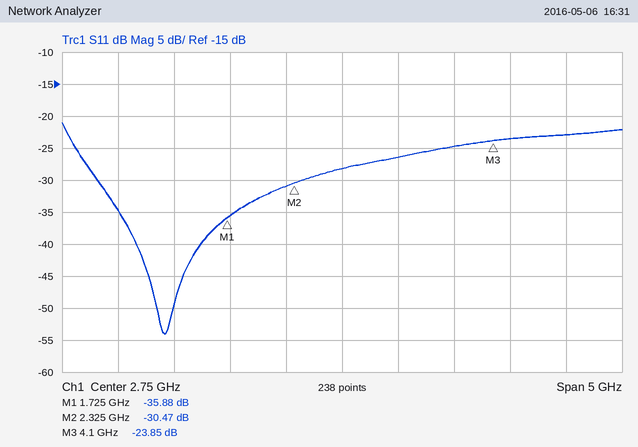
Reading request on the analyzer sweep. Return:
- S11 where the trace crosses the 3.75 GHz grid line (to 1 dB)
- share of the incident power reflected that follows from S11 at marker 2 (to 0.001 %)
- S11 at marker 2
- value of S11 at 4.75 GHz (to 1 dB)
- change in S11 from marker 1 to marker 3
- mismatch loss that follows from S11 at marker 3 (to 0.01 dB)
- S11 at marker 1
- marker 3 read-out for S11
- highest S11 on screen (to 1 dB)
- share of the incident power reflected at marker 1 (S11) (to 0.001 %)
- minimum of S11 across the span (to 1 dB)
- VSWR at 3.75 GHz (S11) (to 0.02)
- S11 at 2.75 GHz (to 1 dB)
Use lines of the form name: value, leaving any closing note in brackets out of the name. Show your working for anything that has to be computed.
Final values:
S11 where the trace crosses the 3.75 GHz grid line: -25 dB
share of the incident power reflected that follows from S11 at marker 2: 10^(-30.47/10) ≈ 0.090 %
S11 at marker 2: -30.47 dB
value of S11 at 4.75 GHz: -23 dB
change in S11 from marker 1 to marker 3: -23.85 − (-35.88) = 12.03 dB
mismatch loss that follows from S11 at marker 3: −10 log10(1 − 10^(-23.85/10)) ≈ 0.02 dB
S11 at marker 1: -35.88 dB
marker 3 read-out for S11: -23.85 dB
highest S11 on screen: -21 dB
share of the incident power reflected at marker 1 (S11): 10^(-35.88/10) ≈ 0.026 %
minimum of S11 across the span: -54 dB
VSWR at 3.75 GHz (S11): |Γ| = 10^(-25/20) = 0.0562; VSWR = (1 + 0.0562)/(1 − 0.0562) ≈ 1.12
S11 at 2.75 GHz: -28 dB
